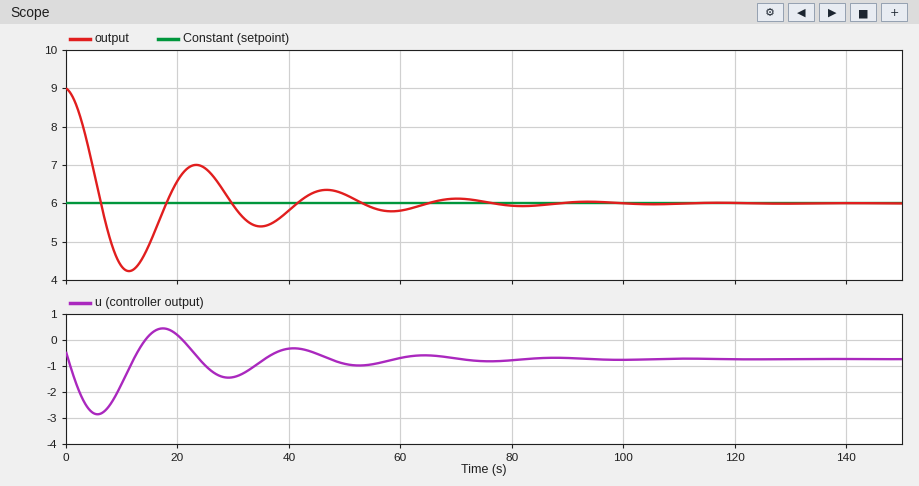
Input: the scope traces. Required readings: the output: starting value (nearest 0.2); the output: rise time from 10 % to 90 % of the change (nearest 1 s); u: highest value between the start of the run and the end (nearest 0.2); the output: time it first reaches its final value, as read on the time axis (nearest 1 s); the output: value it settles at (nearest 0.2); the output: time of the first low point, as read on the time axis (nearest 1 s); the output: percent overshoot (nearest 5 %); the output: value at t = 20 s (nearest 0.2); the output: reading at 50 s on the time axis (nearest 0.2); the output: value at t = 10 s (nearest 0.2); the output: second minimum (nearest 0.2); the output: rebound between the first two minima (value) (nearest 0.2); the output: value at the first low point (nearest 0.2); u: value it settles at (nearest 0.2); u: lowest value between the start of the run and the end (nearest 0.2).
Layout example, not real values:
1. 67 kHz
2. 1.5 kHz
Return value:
1. 9.0
2. 4 s
3. 0.4
4. 6 s
5. 6.0
6. 11 s
7. 60 %
8. 6.6
9. 6.2
10. 4.4
11. 5.4
12. 7.0
13. 4.2
14. -0.8
15. -2.8
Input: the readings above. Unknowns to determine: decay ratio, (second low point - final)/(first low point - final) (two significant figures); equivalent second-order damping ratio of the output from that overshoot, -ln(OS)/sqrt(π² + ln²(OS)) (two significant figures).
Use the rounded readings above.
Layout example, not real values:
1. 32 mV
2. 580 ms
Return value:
1. 0.33
2. 0.16
